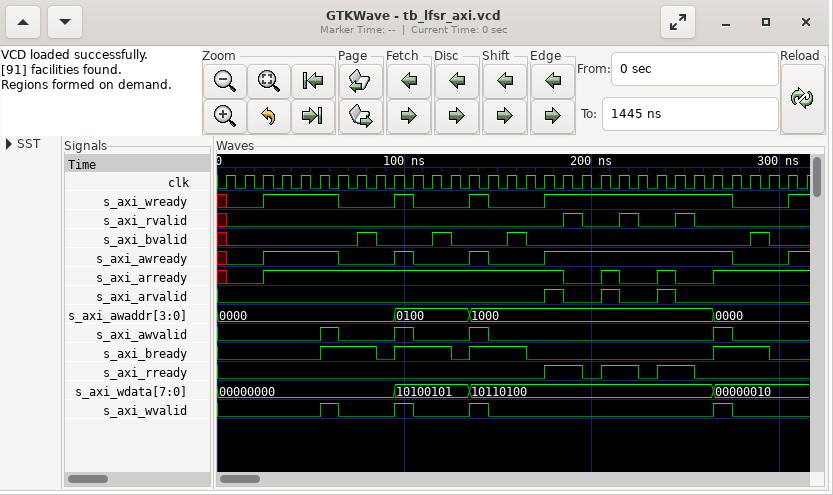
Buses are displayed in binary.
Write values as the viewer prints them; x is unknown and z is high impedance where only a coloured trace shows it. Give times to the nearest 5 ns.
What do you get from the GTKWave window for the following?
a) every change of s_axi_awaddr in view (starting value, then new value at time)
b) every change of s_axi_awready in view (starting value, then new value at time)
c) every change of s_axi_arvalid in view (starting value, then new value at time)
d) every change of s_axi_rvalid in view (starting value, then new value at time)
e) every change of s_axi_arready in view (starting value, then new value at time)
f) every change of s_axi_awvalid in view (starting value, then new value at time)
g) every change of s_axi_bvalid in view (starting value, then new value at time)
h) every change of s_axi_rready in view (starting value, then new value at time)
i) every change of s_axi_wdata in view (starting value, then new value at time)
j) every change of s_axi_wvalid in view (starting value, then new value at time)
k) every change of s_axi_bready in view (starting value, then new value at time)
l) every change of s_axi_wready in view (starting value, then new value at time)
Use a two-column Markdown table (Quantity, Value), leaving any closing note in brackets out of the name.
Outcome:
| Quantity | Value |
|---|---|
| every change of s_axi_awaddr in view | 0000, 0100 at 95 ns, 1000 at 135 ns, 0000 at 265 ns |
| every change of s_axi_awready in view | x, 0 at 5 ns, 1 at 25 ns, 0 at 65 ns, 1 at 95 ns, 0 at 105 ns, 1 at 135 ns, 0 at 145 ns, 1 at 175 ns, 0 at 275 ns, 1 at 305 ns |
| every change of s_axi_arvalid in view | 0, 1 at 175 ns, 0 at 185 ns, 1 at 205 ns, 0 at 215 ns, 1 at 235 ns, 0 at 245 ns |
| every change of s_axi_rvalid in view | x, 0 at 5 ns, 1 at 185 ns, 0 at 195 ns, 1 at 215 ns, 0 at 225 ns, 1 at 245 ns, 0 at 255 ns |
| every change of s_axi_arready in view | x, 0 at 5 ns, 1 at 25 ns, 0 at 185 ns, 1 at 205 ns, 0 at 215 ns, 1 at 235 ns, 0 at 245 ns, 1 at 265 ns |
| every change of s_axi_awvalid in view | 0, 1 at 55 ns, 0 at 65 ns, 1 at 95 ns, 0 at 105 ns, 1 at 135 ns, 0 at 145 ns, 1 at 265 ns, 0 at 275 ns |
| every change of s_axi_bvalid in view | x, 0 at 5 ns, 1 at 75 ns, 0 at 85 ns, 1 at 115 ns, 0 at 125 ns, 1 at 155 ns, 0 at 165 ns, 1 at 285 ns, 0 at 295 ns |
| every change of s_axi_rready in view | 0, 1 at 175 ns, 0 at 195 ns, 1 at 205 ns, 0 at 225 ns, 1 at 235 ns, 0 at 255 ns |
| every change of s_axi_wdata in view | 00000000, 10100101 at 95 ns, 10110100 at 135 ns, 00000010 at 265 ns |
| every change of s_axi_wvalid in view | 0, 1 at 55 ns, 0 at 65 ns, 1 at 95 ns, 0 at 105 ns, 1 at 135 ns, 0 at 145 ns, 1 at 265 ns, 0 at 275 ns |
| every change of s_axi_bready in view | 0, 1 at 55 ns, 0 at 85 ns, 1 at 95 ns, 0 at 125 ns, 1 at 135 ns, 0 at 165 ns, 1 at 265 ns, 0 at 295 ns |
| every change of s_axi_wready in view | x, 0 at 5 ns, 1 at 25 ns, 0 at 65 ns, 1 at 95 ns, 0 at 105 ns, 1 at 135 ns, 0 at 145 ns, 1 at 175 ns, 0 at 275 ns, 1 at 305 ns |
